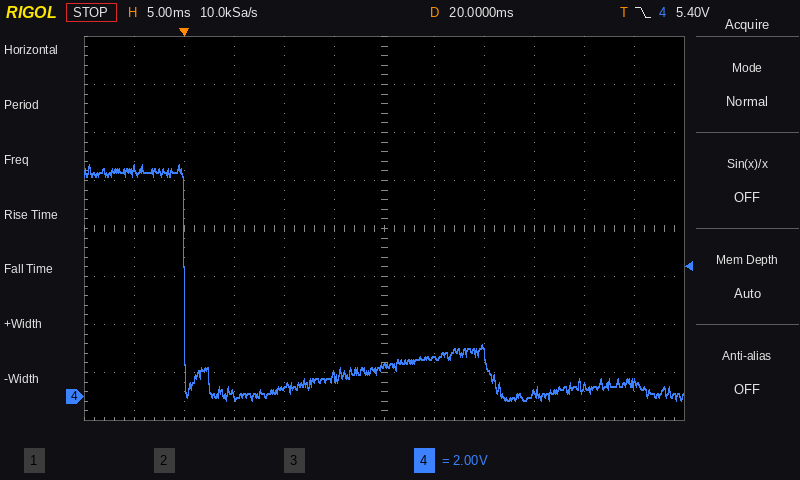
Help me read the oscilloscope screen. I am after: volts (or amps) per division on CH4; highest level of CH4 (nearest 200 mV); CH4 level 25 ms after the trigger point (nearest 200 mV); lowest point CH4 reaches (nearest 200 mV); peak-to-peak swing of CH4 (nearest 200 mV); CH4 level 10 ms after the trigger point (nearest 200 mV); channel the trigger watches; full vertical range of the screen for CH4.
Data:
2 V
9.6 V
1.6 V
-200 mV
9.8 V
400 mV
CH4
16 V
